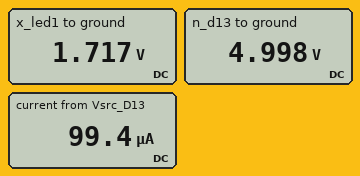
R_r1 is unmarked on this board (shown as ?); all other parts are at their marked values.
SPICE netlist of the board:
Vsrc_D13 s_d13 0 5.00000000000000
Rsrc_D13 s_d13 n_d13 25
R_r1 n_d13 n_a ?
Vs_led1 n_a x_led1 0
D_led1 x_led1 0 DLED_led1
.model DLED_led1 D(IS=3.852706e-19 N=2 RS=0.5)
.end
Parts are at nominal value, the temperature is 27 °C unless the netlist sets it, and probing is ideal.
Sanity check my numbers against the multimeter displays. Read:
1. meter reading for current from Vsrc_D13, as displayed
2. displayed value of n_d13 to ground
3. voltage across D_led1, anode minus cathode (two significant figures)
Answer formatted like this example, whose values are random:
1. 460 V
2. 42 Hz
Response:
1. 99.4 µA
2. 4.998 V
3. 1.7 V
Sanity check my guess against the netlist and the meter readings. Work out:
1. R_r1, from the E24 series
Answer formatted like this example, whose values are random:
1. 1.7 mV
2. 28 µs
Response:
1. 33 kΩ
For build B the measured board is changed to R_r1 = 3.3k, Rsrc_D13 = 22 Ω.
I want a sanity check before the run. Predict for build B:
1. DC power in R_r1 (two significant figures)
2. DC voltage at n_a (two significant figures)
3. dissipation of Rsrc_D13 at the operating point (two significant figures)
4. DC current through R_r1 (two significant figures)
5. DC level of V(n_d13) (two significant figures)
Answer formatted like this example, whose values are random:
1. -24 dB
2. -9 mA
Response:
1. 3.0 mW
2. 1.8 V
3. 20 µW
4. 950 µA
5. 5.0 V
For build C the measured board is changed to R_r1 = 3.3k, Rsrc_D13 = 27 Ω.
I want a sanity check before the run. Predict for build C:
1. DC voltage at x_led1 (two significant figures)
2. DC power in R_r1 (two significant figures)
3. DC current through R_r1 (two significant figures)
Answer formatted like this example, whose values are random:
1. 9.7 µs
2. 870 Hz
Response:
1. 1.8 V
2. 3.0 mW
3. 950 µA
